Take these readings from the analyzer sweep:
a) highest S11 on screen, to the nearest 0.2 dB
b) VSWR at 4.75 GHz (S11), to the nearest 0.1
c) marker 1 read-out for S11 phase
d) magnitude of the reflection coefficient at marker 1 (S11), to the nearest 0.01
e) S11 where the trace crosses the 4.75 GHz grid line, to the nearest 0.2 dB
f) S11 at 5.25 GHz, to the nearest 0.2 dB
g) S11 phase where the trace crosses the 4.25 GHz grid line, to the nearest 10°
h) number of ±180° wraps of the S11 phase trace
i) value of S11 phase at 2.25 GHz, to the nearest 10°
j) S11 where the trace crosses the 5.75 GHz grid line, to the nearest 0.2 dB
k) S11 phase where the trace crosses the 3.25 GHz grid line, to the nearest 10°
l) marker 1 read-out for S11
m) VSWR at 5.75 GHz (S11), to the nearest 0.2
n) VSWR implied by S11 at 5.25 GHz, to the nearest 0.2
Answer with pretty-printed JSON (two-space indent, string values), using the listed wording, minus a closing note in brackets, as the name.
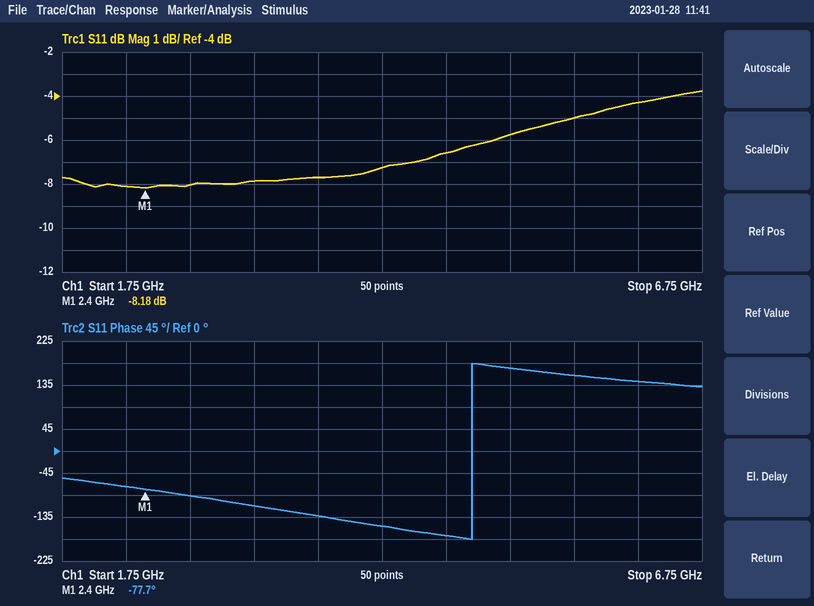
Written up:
{
  "highest S11 on screen, to the nearest 0.2 dB": "-3.8 dB",
  "VSWR at 4.75 GHz (S11), to the nearest 0.1": "2.8",
  "marker 1 read-out for S11 phase": "-77.7°",
  "magnitude of the reflection coefficient at marker 1 (S11), to the nearest 0.01": "0.39",
  "S11 where the trace crosses the 4.75 GHz grid line, to the nearest 0.2 dB": "-6.6 dB",
  "S11 at 5.25 GHz, to the nearest 0.2 dB": "-5.8 dB",
  "S11 phase where the trace crosses the 4.25 GHz grid line, to the nearest 10°": "-150°",
  "number of ±180° wraps of the S11 phase trace": "1",
  "value of S11 phase at 2.25 GHz, to the nearest 10°": "-70°",
  "S11 where the trace crosses the 5.75 GHz grid line, to the nearest 0.2 dB": "-5.0 dB",
  "S11 phase where the trace crosses the 3.25 GHz grid line, to the nearest 10°": "-110°",
  "marker 1 read-out for S11": "-8.18 dB",
  "VSWR at 5.75 GHz (S11), to the nearest 0.2": "3.6",
  "VSWR implied by S11 at 5.25 GHz, to the nearest 0.2": "3.2"
}
